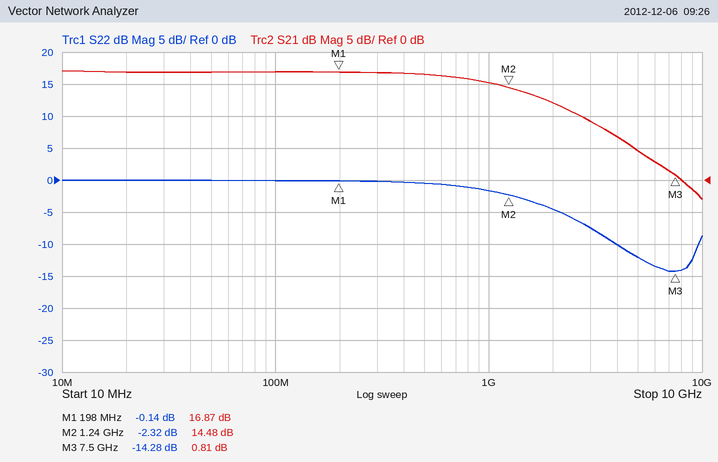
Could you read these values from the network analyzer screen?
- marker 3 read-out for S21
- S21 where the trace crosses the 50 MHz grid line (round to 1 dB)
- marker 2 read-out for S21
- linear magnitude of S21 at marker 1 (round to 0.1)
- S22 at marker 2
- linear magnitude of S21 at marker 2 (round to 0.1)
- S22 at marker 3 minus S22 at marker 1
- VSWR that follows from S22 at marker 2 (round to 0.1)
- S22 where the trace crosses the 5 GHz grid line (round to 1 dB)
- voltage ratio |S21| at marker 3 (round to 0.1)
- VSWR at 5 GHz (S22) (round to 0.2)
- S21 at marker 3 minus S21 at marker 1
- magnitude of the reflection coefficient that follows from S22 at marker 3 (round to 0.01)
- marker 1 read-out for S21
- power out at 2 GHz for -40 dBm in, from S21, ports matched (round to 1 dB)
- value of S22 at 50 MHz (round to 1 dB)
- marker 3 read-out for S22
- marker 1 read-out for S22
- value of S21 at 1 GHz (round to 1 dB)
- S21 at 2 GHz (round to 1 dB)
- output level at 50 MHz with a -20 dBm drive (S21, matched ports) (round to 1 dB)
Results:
0.81 dB
17 dB
14.48 dB
7.0
-2.32 dB
5.3
-14.14 dB
7.5
-12 dB
1.1
1.6
-16.06 dB
0.19
16.87 dB
-28 dBm
0 dB
-14.28 dB
-0.14 dB
15 dB
12 dB
-3 dBm
